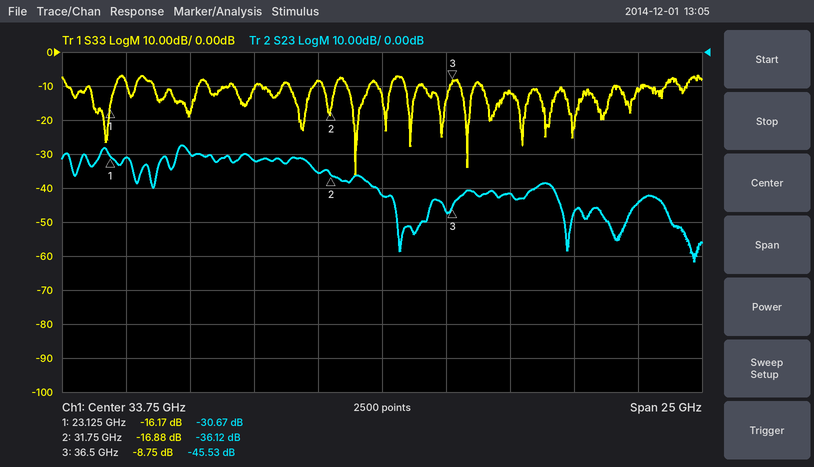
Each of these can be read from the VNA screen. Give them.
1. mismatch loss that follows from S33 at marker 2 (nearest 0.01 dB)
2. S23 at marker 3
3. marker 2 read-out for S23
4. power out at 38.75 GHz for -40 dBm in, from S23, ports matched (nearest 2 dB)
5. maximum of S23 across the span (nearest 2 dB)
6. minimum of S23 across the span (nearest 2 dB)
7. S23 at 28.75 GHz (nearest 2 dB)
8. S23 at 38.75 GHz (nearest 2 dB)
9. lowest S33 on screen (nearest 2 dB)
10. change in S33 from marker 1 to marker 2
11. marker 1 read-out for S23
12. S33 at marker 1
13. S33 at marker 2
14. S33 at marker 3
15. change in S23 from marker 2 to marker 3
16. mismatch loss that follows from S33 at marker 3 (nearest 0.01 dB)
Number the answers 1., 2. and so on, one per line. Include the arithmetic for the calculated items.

1. −10 log10(1 − 10^(-16.88/10)) ≈ 0.09 dB
2. -45.53 dB
3. -36.12 dB
4. -40 dBm + (-42 dB) = -82 dBm
5. -28 dB
6. -62 dB
7. -32 dB
8. -42 dB
9. -36 dB
10. -16.88 − (-16.17) = -0.71 dB
11. -30.67 dB
12. -16.17 dB
13. -16.88 dB
14. -8.75 dB
15. -45.53 − (-36.12) = -9.41 dB
16. −10 log10(1 − 10^(-8.75/10)) ≈ 0.62 dB
